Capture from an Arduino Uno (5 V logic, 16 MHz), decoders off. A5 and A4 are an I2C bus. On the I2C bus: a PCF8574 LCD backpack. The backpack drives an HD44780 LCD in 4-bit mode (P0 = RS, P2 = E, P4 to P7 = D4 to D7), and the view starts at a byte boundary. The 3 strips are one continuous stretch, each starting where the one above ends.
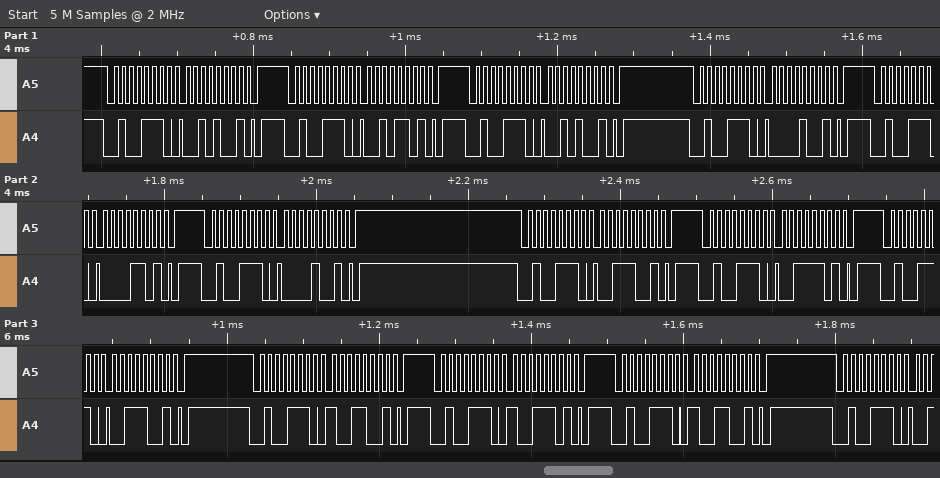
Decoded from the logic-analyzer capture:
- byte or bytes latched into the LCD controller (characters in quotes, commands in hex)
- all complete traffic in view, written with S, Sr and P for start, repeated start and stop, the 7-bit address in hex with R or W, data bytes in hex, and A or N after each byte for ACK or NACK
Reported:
' ' '9'
S 27W A 29 A P S 27W A 2D A P S 27W A 29 A P S 27W A 09 A P S 27W A 0D A P S 27W A 09 A P S 27W A 39 A P S 27W A 3D A P S 27W A 39 A P S 27W A 99 A P S 27W A 9D A P S 27W A 99 A P S 27W A
